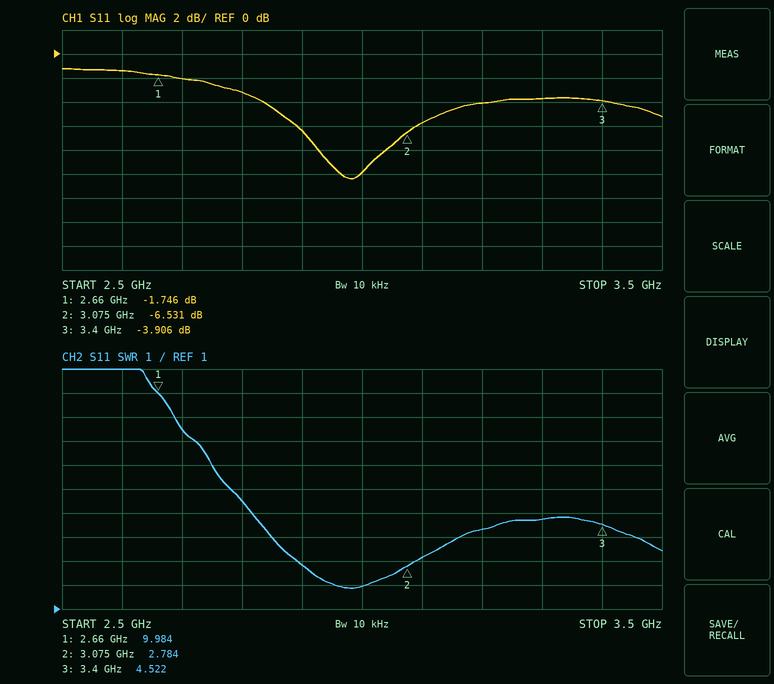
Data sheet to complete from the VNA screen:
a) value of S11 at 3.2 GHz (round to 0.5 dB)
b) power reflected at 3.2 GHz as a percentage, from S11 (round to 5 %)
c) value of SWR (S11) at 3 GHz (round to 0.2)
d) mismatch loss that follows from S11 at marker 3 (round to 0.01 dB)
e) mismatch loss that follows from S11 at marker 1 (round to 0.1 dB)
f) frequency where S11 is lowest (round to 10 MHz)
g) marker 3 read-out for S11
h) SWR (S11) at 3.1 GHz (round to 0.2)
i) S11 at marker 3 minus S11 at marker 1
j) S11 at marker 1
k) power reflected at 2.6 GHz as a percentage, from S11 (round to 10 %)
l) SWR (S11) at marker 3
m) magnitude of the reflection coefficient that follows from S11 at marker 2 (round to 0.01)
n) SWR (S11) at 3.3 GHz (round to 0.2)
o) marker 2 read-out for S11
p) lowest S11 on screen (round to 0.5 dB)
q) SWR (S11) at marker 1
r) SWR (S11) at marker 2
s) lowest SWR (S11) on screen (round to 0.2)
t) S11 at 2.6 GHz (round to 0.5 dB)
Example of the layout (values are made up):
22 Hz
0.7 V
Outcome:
-4.0 dB
40 %
2.0
2.27 dB
4.8 dB
2.98 GHz
-3.906 dB
3.2
-2.160 dB
-1.746 dB
70 %
4.522
0.47
4.8
-6.531 dB
-10.5 dB
9.984
2.784
1.8
-1.5 dB
